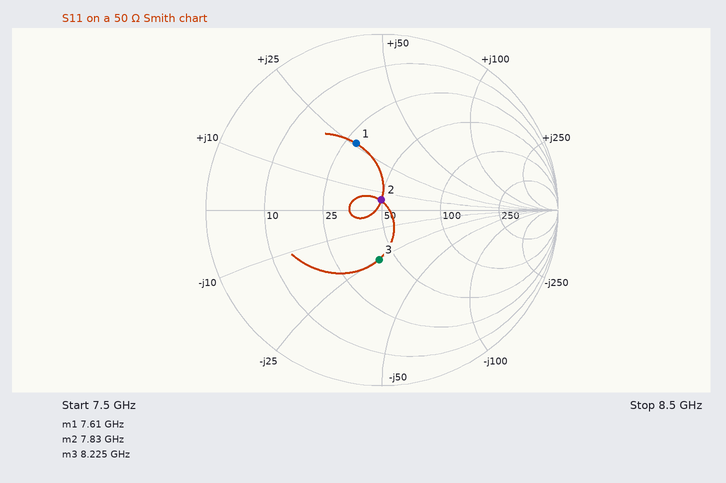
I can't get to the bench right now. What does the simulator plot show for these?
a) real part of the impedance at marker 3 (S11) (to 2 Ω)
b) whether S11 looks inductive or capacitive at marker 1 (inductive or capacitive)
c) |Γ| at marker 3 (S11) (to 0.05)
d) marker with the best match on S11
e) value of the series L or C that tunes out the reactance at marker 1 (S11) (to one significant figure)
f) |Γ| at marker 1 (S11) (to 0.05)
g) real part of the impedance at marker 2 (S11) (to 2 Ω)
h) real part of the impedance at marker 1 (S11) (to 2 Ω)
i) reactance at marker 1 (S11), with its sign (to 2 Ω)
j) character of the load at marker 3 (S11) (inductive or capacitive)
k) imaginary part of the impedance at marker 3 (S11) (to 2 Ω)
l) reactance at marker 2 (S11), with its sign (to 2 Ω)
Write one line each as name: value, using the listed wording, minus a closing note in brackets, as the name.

real part of the impedance at marker 3 (S11): 42 Ω
whether S11 looks inductive or capacitive at marker 1: inductive
|Γ| at marker 3 (S11): 0.30
marker with the best match on S11: marker 2
value of the series L or C that tunes out the reactance at marker 1 (S11): 800 fF
|Γ| at marker 1 (S11): 0.40
real part of the impedance at marker 2 (S11): 50 Ω
real part of the impedance at marker 1 (S11): 28 Ω
reactance at marker 1 (S11), with its sign: +26 Ω
character of the load at marker 3 (S11): capacitive
imaginary part of the impedance at marker 3 (S11): -26 Ω
reactance at marker 2 (S11), with its sign: +6 Ω
